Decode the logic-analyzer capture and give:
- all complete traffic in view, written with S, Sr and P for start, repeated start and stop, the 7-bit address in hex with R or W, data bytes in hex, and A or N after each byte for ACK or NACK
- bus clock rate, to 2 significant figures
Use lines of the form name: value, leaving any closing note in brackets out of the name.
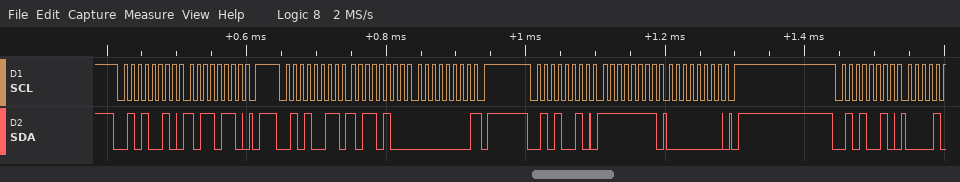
all complete traffic in view, written with S, Sr and P for start, repeated start and stop, the 7-bit address in hex with R or W, data bytes in hex, and A or N after each byte for ACK or NACK: S 29W A B6 A P S 29R A B4 A 00 N P S 29W A FF A 00 A P S 29W A
bus clock rate, to 2 significant figures: 100 kHz
